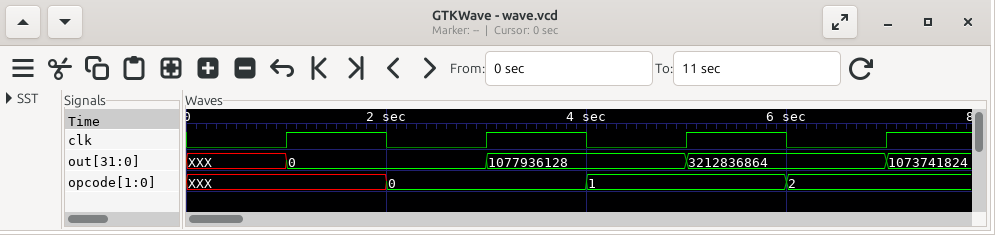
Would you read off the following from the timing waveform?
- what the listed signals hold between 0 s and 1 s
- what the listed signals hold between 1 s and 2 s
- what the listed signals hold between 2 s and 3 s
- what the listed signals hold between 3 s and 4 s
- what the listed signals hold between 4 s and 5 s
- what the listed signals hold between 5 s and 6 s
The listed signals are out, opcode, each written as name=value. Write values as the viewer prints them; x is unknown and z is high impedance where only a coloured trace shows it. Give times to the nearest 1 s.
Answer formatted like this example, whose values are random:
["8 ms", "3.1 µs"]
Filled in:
["out=XXX, opcode=XXX", "out=0, opcode=XXX", "out=0, opcode=0", "out=1077936128, opcode=0", "out=1077936128, opcode=1", "out=3212836864, opcode=1"]
